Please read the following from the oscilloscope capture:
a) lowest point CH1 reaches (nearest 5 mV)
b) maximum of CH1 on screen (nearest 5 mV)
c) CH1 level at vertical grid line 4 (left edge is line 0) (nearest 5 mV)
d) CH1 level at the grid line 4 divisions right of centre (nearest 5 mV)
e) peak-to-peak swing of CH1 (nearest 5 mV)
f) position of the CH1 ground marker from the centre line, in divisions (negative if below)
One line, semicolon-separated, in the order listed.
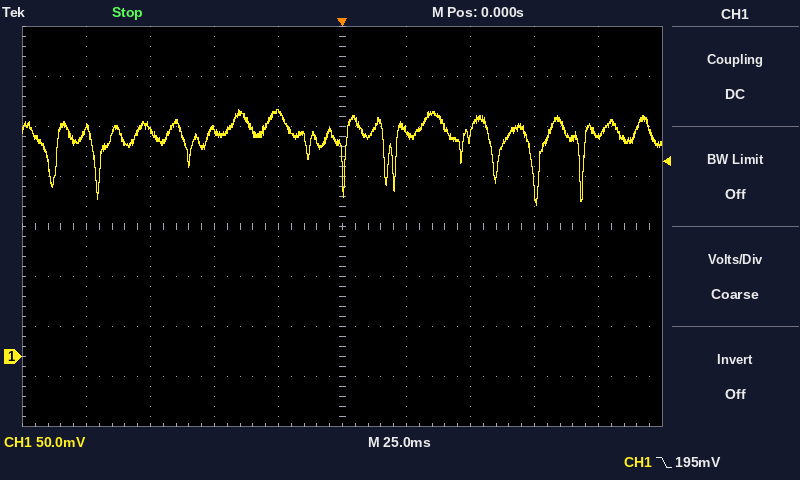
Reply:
150 mV; 245 mV; 245 mV; 220 mV; 95 mV; -2.6 div
